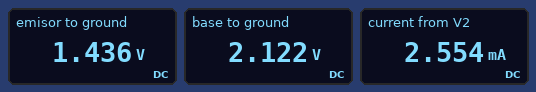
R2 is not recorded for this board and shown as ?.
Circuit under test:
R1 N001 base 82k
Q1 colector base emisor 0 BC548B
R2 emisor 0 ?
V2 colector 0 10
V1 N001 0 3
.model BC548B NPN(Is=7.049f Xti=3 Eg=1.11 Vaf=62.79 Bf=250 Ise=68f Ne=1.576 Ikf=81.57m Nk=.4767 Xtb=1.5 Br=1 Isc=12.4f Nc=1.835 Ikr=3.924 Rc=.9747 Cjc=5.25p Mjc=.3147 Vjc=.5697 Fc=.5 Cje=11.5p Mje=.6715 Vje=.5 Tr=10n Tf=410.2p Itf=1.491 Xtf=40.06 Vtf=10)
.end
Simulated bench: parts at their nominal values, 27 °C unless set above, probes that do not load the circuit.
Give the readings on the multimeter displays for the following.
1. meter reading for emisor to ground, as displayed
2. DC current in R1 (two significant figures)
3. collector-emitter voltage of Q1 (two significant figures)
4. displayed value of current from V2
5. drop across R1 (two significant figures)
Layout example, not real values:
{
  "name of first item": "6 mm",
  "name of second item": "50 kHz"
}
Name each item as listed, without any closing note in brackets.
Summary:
{
  "meter reading for emisor to ground, as displayed": "1.436 V",
  "DC current in R1": "11 µA",
  "collector-emitter voltage of Q1": "8.6 V",
  "displayed value of current from V2": "2.554 mA",
  "drop across R1": "880 mV"
}
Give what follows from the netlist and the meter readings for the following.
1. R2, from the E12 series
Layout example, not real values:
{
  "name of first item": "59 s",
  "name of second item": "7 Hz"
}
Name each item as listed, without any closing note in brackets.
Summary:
{
  "R2, from the E12 series": "560 Ω"
}
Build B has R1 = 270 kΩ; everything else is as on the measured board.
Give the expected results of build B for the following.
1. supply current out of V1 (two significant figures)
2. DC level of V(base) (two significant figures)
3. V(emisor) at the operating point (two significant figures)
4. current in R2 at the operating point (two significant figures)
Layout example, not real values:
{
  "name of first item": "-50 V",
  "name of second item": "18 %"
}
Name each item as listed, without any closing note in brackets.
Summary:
{
  "supply current out of V1": "5.8 µA",
  "DC level of V(base)": "1.4 V",
  "V(emisor) at the operating point": "770 mV",
  "current in R2 at the operating point": "1.4 mA"
}
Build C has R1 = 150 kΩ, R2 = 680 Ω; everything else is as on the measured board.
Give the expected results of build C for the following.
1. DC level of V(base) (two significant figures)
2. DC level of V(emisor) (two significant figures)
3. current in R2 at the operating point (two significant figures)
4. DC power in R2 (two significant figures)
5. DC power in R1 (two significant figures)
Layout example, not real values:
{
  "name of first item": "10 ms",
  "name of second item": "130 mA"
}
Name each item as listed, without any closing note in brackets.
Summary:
{
  "DC level of V(base)": "1.9 V",
  "DC level of V(emisor)": "1.2 V",
  "current in R2 at the operating point": "1.8 mA",
  "DC power in R2": "2.1 mW",
  "DC power in R1": "8.3 µW"
}
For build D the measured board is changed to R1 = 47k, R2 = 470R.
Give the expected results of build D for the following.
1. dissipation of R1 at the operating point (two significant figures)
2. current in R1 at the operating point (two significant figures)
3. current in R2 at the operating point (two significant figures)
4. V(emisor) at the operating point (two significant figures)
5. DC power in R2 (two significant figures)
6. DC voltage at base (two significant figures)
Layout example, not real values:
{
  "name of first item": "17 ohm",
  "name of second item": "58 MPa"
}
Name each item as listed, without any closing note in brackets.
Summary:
{
  "dissipation of R1 at the operating point": "9.8 µW",
  "current in R1 at the operating point": "14 µA",
  "current in R2 at the operating point": "3.5 mA",
  "V(emisor) at the operating point": "1.6 V",
  "DC power in R2": "5.6 mW",
  "DC voltage at base": "2.3 V"
}
